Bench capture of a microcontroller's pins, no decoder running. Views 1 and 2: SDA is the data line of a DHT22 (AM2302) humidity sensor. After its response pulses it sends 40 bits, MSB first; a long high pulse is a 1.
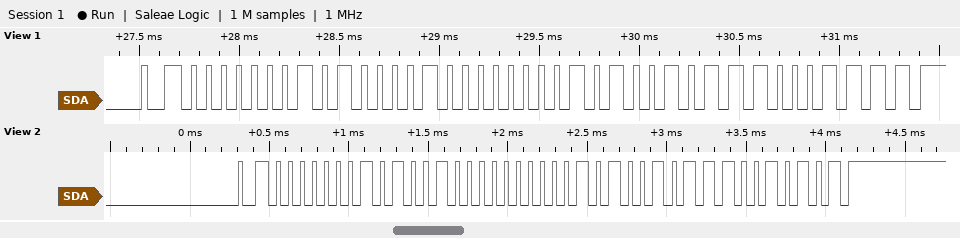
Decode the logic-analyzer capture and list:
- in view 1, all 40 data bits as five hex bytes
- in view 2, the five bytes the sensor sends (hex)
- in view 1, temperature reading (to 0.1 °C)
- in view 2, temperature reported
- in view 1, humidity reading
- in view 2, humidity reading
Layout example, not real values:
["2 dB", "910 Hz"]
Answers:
["01 42 01 4B 8F", "01 48 01 4B 95", "33.1 °C", "33.1 °C", "32.2 %", "32.8 %"]
